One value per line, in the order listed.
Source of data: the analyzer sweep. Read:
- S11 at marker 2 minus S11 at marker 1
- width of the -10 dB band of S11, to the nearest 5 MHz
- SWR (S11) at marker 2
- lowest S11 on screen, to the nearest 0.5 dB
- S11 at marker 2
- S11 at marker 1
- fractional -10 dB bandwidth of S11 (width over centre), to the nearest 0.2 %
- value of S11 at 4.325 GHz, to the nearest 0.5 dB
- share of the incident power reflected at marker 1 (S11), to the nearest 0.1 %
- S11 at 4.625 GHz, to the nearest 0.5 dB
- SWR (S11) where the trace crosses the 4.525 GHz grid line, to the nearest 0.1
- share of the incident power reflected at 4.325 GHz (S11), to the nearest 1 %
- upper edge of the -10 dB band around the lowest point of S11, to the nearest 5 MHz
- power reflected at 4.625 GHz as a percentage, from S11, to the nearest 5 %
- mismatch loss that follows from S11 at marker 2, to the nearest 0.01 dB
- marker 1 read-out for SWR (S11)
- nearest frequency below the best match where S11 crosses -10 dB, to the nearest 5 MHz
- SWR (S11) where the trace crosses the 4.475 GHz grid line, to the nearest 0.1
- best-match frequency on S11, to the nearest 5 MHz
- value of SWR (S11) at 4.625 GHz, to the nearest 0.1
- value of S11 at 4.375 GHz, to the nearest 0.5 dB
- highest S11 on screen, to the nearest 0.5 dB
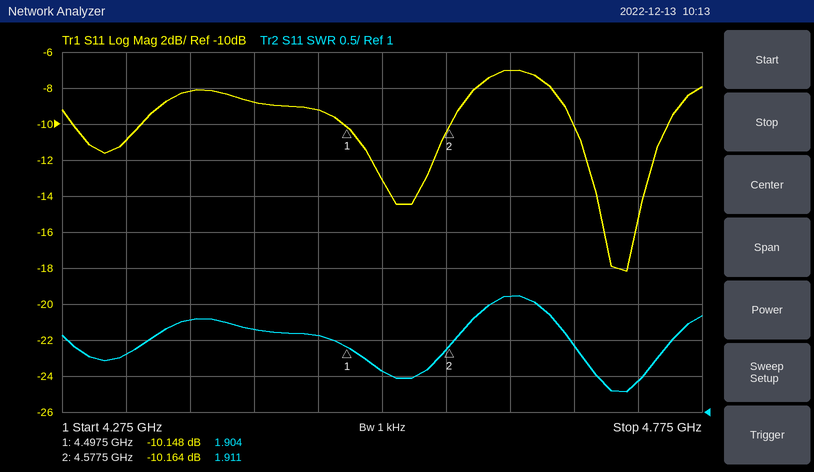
-0.016 dB
75 MHz
1.911
-18.0 dB
-10.164 dB
-10.148 dB
1.6 %
-11.0 dB
9.7 %
-7.0 dB
1.6
8 %
4.750 GHz
20 %
0.44 dB
1.904
4.675 GHz
2.1
4.715 GHz
2.6
-8.0 dB
-7.0 dB
